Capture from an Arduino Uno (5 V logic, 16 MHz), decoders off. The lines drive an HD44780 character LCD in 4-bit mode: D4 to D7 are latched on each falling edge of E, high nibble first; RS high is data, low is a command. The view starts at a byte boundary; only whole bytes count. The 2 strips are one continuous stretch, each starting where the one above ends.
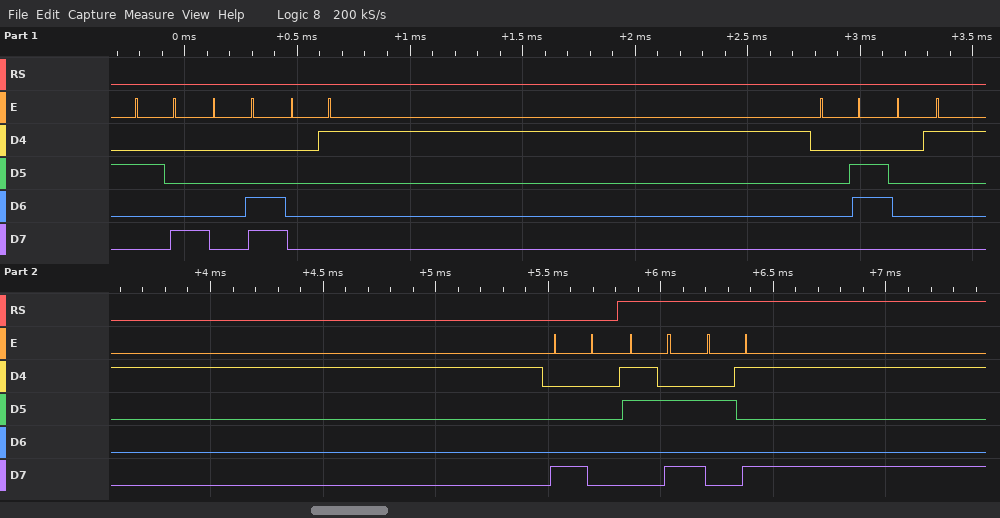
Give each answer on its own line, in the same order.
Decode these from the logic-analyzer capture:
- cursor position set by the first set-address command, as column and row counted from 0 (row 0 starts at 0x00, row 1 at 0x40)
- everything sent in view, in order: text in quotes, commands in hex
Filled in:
column 0, row 0
0x28 0x0C 0x01 0x06 0x01 0x80 ":)"
